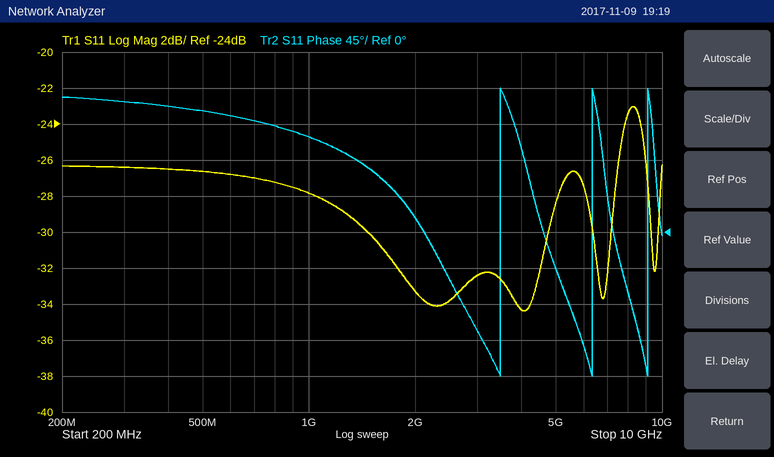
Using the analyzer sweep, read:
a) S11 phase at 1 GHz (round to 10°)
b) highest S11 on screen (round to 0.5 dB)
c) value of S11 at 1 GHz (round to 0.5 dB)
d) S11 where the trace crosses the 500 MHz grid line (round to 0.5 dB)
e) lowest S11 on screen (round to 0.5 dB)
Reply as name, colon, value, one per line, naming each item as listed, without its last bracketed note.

S11 phase at 1 GHz: 120°
highest S11 on screen: -23.0 dB
value of S11 at 1 GHz: -28.0 dB
S11 where the trace crosses the 500 MHz grid line: -26.5 dB
lowest S11 on screen: -34.5 dB
